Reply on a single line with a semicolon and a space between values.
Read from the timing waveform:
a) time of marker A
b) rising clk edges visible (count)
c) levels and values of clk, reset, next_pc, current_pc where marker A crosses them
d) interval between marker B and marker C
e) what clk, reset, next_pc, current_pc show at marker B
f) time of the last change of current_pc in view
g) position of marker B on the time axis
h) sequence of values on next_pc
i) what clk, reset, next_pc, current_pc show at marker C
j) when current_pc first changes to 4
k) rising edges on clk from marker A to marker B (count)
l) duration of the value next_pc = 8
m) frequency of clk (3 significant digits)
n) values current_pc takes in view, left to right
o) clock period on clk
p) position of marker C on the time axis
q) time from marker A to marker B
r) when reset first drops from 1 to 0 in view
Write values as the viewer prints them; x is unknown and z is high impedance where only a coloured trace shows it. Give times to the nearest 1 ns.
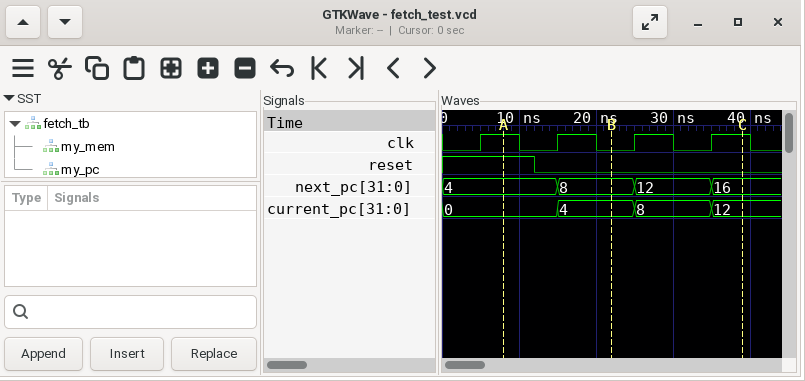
8 ns; 4; clk=1, reset=1, next_pc=4, current_pc=0; 17 ns; clk=0, reset=0, next_pc=8, current_pc=4; 35 ns; 22 ns; 4, 8, 12, 16; clk=1, reset=0, next_pc=16, current_pc=12; 15 ns; 1; 10 ns; 100 MHz; 0, 4, 8, 12; 10 ns; 39 ns; 14 ns; 12 ns
